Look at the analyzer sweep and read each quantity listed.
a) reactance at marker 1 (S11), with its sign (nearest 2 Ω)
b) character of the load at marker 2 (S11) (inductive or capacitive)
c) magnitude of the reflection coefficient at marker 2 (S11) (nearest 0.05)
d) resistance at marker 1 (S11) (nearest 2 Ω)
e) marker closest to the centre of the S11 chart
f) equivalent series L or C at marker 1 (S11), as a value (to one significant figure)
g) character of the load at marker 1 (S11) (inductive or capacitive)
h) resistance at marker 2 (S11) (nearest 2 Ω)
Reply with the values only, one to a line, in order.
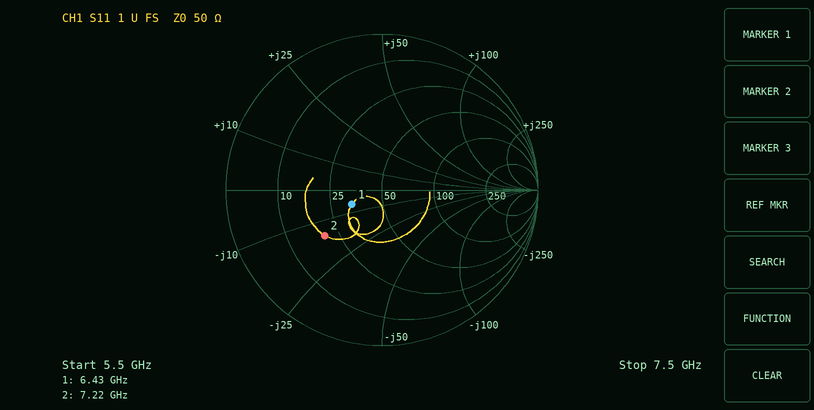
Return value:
-6 Ω
capacitive
0.45
34 Ω
marker 1
4 pF
capacitive
20 Ω
